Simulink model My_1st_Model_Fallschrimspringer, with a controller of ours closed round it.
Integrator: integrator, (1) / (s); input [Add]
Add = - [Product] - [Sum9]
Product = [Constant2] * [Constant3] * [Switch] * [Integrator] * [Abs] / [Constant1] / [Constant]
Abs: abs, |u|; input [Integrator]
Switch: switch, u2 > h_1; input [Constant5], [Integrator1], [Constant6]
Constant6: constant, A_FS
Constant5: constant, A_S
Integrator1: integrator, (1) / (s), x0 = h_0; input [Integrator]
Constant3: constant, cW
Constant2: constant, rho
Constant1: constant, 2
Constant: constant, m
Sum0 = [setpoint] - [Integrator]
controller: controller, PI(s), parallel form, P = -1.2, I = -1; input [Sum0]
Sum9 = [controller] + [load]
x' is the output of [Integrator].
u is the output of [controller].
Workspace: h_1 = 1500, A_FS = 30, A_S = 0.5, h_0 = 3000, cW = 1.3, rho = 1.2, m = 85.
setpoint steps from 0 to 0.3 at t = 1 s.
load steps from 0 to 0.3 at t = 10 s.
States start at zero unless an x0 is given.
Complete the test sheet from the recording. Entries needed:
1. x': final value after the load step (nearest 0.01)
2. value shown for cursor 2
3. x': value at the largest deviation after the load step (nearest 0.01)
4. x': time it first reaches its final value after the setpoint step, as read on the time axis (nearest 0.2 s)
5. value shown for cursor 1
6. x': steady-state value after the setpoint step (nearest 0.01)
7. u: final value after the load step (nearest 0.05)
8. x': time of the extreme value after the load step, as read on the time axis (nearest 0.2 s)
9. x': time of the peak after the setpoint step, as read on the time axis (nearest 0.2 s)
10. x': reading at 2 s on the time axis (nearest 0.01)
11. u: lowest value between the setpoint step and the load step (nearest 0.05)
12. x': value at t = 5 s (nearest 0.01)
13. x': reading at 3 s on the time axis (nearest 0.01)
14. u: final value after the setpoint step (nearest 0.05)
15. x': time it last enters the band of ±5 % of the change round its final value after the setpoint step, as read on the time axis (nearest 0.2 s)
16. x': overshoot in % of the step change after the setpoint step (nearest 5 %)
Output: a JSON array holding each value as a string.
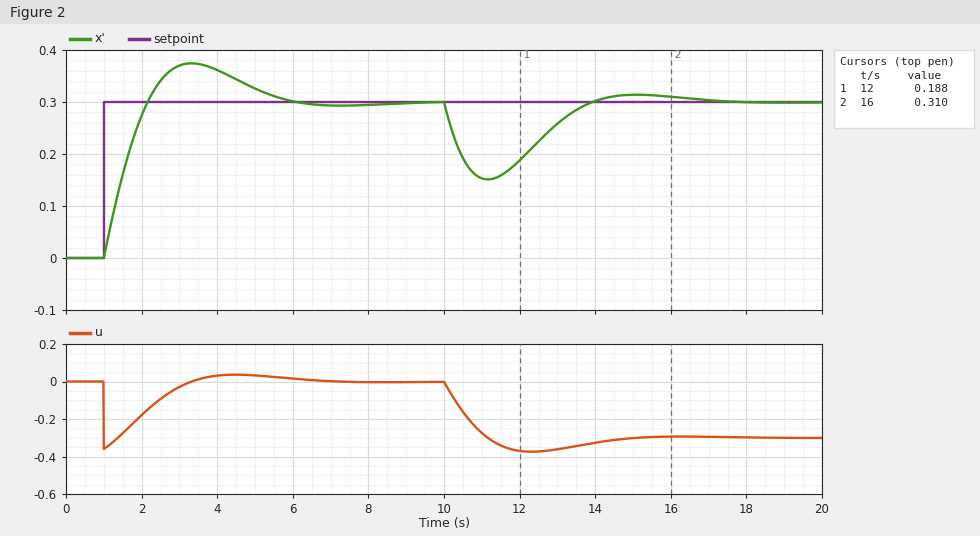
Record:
["0.30", "0.310", "0.15", "2.2 s", "0.188", "0.30", "-0.30", "11.2 s", "3.4 s", "0.27", "-0.35", "0.33", "0.37", "0.00", "5.4 s", "25 %"]
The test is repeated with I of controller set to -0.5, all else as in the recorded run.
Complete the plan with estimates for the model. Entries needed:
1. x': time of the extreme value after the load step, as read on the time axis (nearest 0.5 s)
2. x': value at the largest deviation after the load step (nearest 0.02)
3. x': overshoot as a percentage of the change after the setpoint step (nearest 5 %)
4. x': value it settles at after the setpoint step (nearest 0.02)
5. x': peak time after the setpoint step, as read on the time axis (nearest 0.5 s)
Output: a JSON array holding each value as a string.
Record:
["11.5 s", "0.12", "15 %", "0.30", "4.0 s"]
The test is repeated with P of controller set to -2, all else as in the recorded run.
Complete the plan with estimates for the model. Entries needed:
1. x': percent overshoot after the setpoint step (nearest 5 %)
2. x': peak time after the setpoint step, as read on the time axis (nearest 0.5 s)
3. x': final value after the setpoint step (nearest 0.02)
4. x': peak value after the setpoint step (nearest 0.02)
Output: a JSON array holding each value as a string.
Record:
["15 %", "3.0 s", "0.30", "0.34"]
